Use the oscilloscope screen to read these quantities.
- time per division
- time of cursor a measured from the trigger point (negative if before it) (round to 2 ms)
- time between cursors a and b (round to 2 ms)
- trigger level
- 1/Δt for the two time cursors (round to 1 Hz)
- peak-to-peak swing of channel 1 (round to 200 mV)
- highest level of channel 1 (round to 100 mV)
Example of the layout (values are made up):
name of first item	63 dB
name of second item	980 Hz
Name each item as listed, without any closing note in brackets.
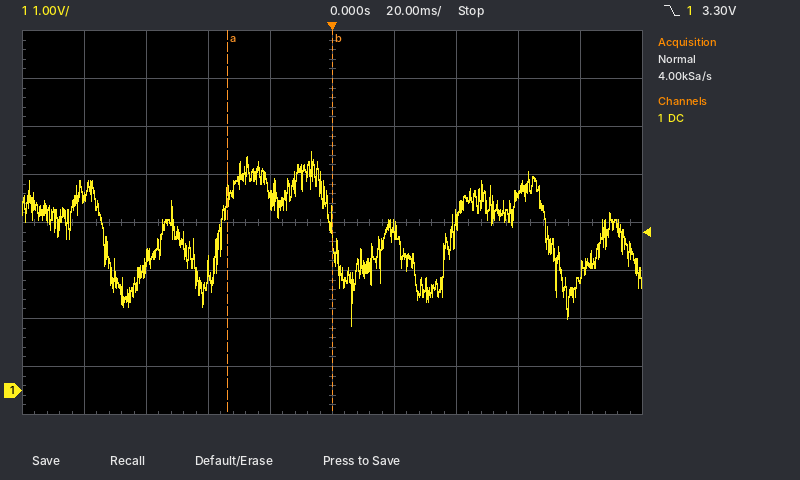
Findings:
time per division	20 ms
time of cursor a measured from the trigger point (negative if before it)	-34 ms
time between cursors a and b	34 ms
trigger level	3.30 V
1/Δt for the two time cursors	29 Hz
peak-to-peak swing of channel 1	3.6 V
highest level of channel 1	5.0 V
